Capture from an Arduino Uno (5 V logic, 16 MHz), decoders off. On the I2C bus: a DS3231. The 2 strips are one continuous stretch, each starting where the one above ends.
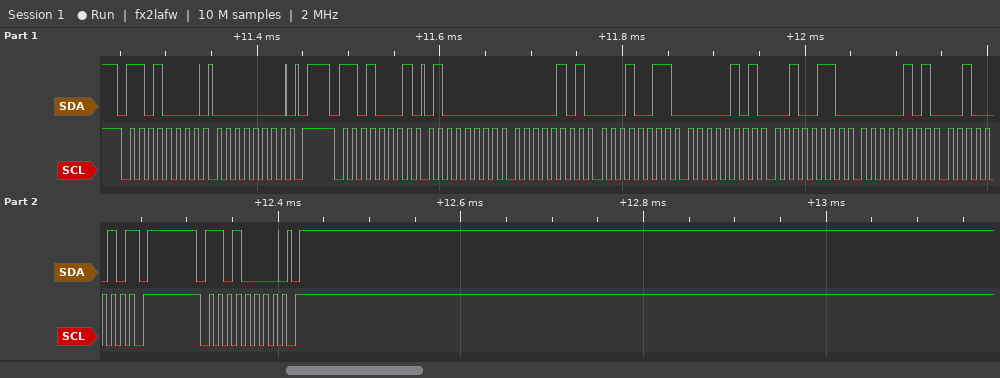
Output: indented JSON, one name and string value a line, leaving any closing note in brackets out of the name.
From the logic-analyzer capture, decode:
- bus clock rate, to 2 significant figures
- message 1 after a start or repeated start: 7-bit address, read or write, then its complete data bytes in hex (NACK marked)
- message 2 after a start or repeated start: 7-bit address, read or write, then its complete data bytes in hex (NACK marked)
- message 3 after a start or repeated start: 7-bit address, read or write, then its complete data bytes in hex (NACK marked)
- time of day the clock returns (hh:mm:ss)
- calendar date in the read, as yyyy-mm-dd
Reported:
{
  "bus clock rate, to 2 significant figures": "100 kHz",
  "message 1 after a start or repeated start: 7-bit address, read or write, then its complete data bytes in hex": "0x68 write: 00",
  "message 2 after a start or repeated start: 7-bit address, read or write, then its complete data bytes in hex": "0x68 read: 40 05 13 05 26 05 22 NACK",
  "message 3 after a start or repeated start: 7-bit address, read or write, then its complete data bytes in hex": "0x68 write",
  "time of day the clock returns": "13:05:40",
  "calendar date in the read, as yyyy-mm-dd": "2022-05-26"
}
